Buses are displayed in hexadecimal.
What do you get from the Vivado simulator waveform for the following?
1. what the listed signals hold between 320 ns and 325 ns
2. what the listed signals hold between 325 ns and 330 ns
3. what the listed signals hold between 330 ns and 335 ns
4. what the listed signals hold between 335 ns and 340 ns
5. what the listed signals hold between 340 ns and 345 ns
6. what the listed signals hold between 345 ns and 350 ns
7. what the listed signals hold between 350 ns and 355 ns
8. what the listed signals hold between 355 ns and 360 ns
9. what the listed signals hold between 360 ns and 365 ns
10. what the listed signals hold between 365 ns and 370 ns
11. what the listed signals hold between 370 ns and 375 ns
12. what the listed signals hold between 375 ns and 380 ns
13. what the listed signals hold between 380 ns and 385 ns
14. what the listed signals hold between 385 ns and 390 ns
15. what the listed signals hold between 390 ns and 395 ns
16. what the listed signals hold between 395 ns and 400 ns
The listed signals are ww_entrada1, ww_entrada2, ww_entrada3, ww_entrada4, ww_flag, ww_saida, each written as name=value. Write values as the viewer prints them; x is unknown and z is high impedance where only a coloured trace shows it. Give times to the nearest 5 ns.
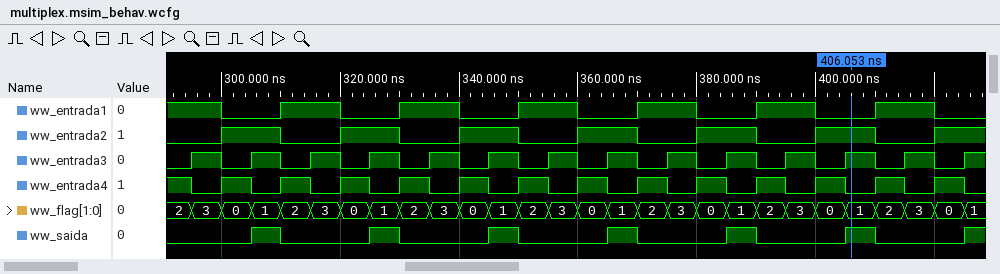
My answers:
ww_entrada1=0, ww_entrada2=1, ww_entrada3=0, ww_entrada4=1, ww_flag=0, ww_saida=0
ww_entrada1=0, ww_entrada2=1, ww_entrada3=1, ww_entrada4=0, ww_flag=1, ww_saida=1
ww_entrada1=1, ww_entrada2=0, ww_entrada3=0, ww_entrada4=1, ww_flag=2, ww_saida=0
ww_entrada1=1, ww_entrada2=0, ww_entrada3=1, ww_entrada4=0, ww_flag=3, ww_saida=0
ww_entrada1=0, ww_entrada2=1, ww_entrada3=0, ww_entrada4=1, ww_flag=0, ww_saida=0
ww_entrada1=0, ww_entrada2=1, ww_entrada3=1, ww_entrada4=0, ww_flag=1, ww_saida=1
ww_entrada1=1, ww_entrada2=0, ww_entrada3=0, ww_entrada4=1, ww_flag=2, ww_saida=0
ww_entrada1=1, ww_entrada2=0, ww_entrada3=1, ww_entrada4=0, ww_flag=3, ww_saida=0
ww_entrada1=0, ww_entrada2=1, ww_entrada3=0, ww_entrada4=1, ww_flag=0, ww_saida=0
ww_entrada1=0, ww_entrada2=1, ww_entrada3=1, ww_entrada4=0, ww_flag=1, ww_saida=1
ww_entrada1=1, ww_entrada2=0, ww_entrada3=0, ww_entrada4=1, ww_flag=2, ww_saida=0
ww_entrada1=1, ww_entrada2=0, ww_entrada3=1, ww_entrada4=0, ww_flag=3, ww_saida=0
ww_entrada1=0, ww_entrada2=1, ww_entrada3=0, ww_entrada4=1, ww_flag=0, ww_saida=0
ww_entrada1=0, ww_entrada2=1, ww_entrada3=1, ww_entrada4=0, ww_flag=1, ww_saida=1
ww_entrada1=1, ww_entrada2=0, ww_entrada3=0, ww_entrada4=1, ww_flag=2, ww_saida=0
ww_entrada1=1, ww_entrada2=0, ww_entrada3=1, ww_entrada4=0, ww_flag=3, ww_saida=0
